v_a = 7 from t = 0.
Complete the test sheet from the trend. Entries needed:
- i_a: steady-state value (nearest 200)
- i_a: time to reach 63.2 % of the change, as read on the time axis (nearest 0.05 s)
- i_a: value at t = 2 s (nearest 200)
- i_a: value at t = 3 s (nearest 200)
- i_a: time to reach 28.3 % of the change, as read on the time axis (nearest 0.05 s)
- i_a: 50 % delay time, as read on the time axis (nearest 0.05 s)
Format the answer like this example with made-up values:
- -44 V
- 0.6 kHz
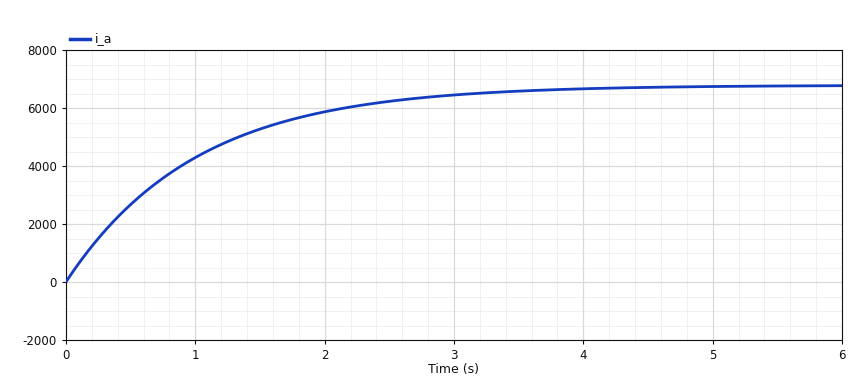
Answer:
- 6800
- 1.00 s
- 5800
- 6400
- 0.35 s
- 0.70 s
